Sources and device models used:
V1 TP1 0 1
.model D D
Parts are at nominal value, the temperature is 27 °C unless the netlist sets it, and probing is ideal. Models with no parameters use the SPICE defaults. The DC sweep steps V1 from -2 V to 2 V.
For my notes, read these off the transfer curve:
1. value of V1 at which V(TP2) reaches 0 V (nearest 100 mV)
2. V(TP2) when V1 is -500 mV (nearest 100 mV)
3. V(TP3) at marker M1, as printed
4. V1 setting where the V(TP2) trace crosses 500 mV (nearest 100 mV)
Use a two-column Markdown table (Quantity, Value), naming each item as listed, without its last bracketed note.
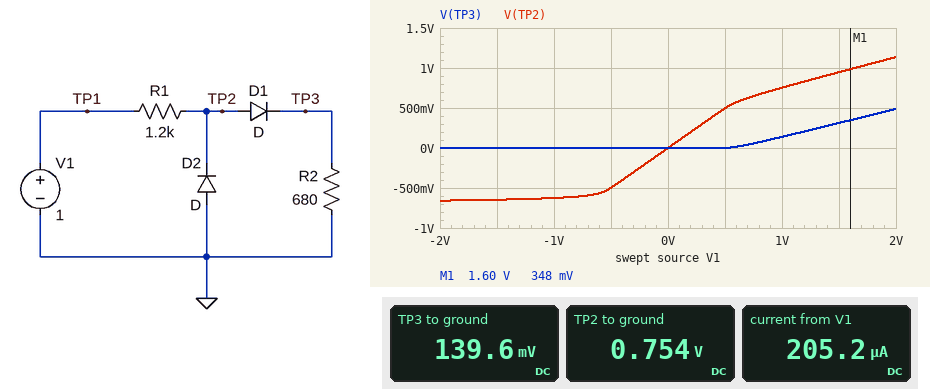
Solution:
| Quantity | Value |
|---|---|
| value of V1 at which V(TP2) reaches 0 V | 0 V |
| V(TP2) when V1 is -500 mV | -500 mV |
| V(TP3) at marker M1, as printed | 348 mV |
| V1 setting where the V(TP2) trace crosses 500 mV | 500 mV |
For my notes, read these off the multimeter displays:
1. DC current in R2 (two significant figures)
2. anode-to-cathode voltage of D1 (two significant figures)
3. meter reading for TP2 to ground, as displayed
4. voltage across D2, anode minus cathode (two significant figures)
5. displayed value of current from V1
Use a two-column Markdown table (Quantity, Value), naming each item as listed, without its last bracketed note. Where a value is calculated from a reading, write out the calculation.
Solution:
| Quantity | Value |
|---|---|
| DC current in R2 | (139.6 mV) / 680 Ω = 210 µA |
| anode-to-cathode voltage of D1 | 754 mV - 139.6 mV = 610 mV |
| meter reading for TP2 to ground, as displayed | 0.754 V |
| voltage across D2, anode minus cathode | 0 V - 754 mV = -750 mV |
| displayed value of current from V1 | 205.2 µA |
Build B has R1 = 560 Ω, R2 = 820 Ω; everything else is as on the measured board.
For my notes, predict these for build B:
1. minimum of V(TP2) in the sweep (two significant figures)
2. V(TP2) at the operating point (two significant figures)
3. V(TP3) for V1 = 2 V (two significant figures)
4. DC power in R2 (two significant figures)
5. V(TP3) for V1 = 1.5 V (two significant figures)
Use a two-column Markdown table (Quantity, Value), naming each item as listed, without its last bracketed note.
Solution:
| Quantity | Value |
|---|---|
| minimum of V(TP2) in the sweep | -680 mV |
| V(TP2) at the operating point | 850 mV |
| V(TP3) for V1 = 2 V | 800 mV |
| DC power in R2 | 62 µW |
| V(TP3) for V1 = 1.5 V | 510 mV |
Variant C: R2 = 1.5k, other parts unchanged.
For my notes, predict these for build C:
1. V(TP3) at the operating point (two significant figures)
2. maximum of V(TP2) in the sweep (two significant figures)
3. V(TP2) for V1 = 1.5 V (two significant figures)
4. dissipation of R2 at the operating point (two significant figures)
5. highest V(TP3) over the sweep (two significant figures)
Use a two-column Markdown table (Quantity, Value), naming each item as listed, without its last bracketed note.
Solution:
| Quantity | Value |
|---|---|
| V(TP3) at the operating point | 220 mV |
| maximum of V(TP2) in the sweep | 1.4 V |
| V(TP2) for V1 = 1.5 V | 1.1 V |
| dissipation of R2 at the operating point | 32 µW |
| highest V(TP3) over the sweep | 760 mV |
